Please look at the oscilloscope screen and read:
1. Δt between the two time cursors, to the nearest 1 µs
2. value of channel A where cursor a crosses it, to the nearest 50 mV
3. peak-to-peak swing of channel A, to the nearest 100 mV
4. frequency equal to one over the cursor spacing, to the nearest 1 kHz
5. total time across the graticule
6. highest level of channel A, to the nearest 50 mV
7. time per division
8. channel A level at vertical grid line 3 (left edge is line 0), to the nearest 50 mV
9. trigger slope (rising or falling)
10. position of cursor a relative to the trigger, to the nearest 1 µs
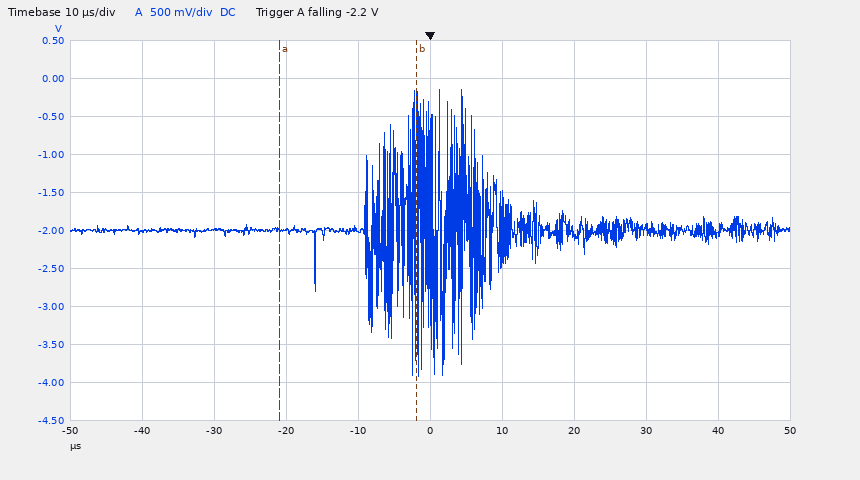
19 µs
-2.00 V
3.80 V
53 kHz
100 µs
-150 mV
10 µs
-2.00 V
falling
-21 µs
